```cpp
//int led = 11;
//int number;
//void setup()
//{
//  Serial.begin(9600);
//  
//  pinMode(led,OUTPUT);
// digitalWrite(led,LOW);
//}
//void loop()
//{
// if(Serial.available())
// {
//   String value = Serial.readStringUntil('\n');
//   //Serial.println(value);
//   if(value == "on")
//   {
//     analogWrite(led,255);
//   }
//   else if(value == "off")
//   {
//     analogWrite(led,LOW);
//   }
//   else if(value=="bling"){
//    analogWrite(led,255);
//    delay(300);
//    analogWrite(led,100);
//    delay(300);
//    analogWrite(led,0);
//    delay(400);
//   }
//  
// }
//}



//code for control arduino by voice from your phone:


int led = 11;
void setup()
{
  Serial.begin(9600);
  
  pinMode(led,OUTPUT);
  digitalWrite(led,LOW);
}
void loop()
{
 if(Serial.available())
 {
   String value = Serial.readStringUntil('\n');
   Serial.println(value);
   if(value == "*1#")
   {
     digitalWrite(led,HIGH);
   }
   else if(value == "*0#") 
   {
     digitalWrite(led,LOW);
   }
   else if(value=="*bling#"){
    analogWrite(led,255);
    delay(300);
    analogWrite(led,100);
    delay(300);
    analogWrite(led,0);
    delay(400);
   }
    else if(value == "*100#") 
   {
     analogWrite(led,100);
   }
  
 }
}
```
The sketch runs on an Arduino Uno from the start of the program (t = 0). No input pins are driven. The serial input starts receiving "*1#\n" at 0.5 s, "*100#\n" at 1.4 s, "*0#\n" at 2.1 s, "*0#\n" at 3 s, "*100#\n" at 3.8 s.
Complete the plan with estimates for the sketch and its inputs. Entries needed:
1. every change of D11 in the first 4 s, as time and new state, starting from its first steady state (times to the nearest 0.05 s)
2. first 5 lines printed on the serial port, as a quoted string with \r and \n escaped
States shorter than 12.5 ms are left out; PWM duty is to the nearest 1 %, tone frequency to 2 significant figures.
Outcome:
0 s low; 0.5 s high; 1.4 s PWM 39 %; 2.1 s low; 3.8 s PWM 39 %
"*1#\r\n*100#\r\n*0#\r\n*0#\r\n*100#\r\n"
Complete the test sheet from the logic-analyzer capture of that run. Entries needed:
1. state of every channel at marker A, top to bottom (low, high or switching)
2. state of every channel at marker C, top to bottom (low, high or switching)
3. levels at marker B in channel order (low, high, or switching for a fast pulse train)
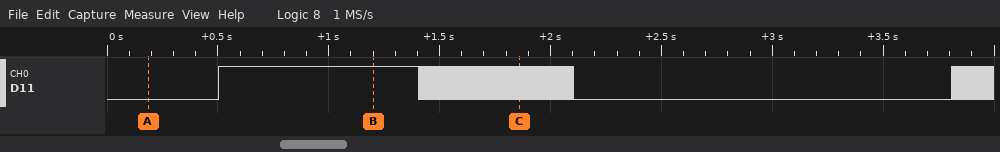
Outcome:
D11 low
D11 switching
D11 high
